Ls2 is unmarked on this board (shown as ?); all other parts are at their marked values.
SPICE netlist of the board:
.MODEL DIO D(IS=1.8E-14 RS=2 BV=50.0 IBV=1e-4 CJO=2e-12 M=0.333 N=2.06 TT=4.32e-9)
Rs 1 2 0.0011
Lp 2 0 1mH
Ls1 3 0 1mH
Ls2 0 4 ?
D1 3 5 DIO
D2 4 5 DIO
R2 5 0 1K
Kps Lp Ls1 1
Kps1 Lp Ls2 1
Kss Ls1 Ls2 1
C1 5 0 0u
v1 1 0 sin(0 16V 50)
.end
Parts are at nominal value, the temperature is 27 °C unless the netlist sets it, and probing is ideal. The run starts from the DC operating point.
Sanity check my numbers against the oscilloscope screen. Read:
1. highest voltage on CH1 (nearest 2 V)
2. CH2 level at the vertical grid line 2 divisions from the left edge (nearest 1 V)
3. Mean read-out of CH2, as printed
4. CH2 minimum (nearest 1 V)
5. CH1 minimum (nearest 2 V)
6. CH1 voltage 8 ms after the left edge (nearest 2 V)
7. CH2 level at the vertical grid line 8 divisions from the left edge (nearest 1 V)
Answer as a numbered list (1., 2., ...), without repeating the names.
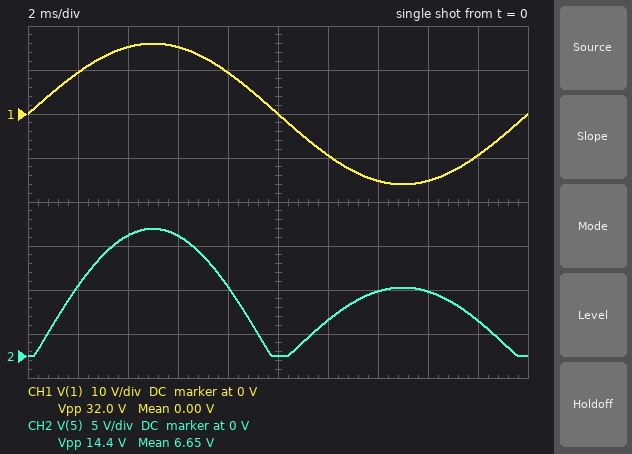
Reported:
1. 16 V
2. 14 V
3. 6.65 V
4. 0 V
5. -16 V
6. 10 V
7. 7 V
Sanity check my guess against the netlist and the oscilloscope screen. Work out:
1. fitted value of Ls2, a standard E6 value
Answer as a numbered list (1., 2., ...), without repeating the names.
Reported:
1. 330 µH
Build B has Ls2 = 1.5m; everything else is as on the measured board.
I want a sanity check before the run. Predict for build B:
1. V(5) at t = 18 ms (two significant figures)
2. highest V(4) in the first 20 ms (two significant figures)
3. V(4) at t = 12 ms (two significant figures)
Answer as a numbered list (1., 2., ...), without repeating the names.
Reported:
1. 10 V
2. 20 V
3. 12 V
